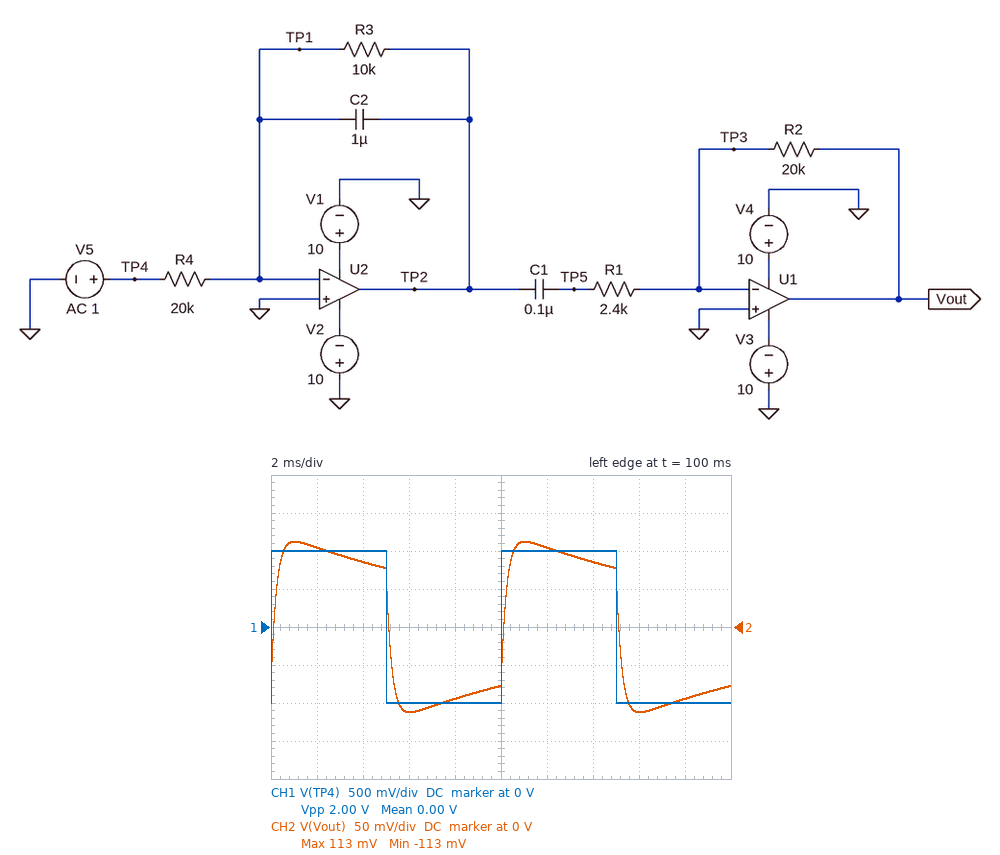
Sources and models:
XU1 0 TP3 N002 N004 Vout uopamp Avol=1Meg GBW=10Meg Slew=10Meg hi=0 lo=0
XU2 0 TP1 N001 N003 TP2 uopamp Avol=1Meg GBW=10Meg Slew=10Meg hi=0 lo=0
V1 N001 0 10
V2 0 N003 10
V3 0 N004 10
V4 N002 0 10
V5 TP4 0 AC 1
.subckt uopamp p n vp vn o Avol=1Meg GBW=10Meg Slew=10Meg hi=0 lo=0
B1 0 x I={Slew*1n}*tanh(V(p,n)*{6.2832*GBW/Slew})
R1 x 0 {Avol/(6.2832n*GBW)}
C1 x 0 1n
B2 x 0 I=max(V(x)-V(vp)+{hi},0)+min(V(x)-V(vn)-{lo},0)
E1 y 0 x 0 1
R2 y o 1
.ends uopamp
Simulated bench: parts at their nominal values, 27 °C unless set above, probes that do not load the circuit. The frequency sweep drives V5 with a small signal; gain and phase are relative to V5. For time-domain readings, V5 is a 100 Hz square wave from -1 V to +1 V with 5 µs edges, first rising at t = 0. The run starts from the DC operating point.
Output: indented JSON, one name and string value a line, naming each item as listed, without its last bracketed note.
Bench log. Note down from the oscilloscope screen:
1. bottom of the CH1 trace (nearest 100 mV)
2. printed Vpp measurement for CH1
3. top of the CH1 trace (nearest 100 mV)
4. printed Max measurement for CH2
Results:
{
  "bottom of the CH1 trace": "-1.0 V",
  "printed Vpp measurement for CH1": "2.00 V",
  "top of the CH1 trace": "1.0 V",
  "printed Max measurement for CH2": "113 mV"
}
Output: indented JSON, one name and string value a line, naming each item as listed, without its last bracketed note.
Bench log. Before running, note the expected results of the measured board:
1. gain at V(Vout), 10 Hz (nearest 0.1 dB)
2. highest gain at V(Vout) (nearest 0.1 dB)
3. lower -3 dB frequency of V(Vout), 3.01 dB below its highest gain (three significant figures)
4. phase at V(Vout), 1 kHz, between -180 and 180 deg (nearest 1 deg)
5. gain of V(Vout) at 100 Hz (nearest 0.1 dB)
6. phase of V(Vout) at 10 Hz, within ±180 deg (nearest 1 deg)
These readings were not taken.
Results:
{
  "gain at V(Vout), 10 Hz": "-25.5 dB",
  "highest gain at V(Vout)": "-20.2 dB",
  "lower -3 dB frequency of V(Vout), 3.01 dB below its highest gain": "15.2 Hz",
  "phase at V(Vout), 1 kHz, between -180 and 180 deg": "-56 deg",
  "gain of V(Vout) at 100 Hz": "-20.2 dB",
  "phase of V(Vout) at 10 Hz, within ±180 deg": "57 deg"
}
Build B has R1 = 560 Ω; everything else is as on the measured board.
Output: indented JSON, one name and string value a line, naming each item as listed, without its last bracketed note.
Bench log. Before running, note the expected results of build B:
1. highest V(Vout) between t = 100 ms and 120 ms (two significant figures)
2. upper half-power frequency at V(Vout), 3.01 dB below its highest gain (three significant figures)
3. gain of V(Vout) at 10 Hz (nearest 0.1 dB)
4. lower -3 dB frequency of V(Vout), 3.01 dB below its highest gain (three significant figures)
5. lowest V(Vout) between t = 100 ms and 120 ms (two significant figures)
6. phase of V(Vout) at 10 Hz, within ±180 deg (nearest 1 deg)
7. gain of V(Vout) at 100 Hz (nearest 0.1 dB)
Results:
{
  "highest V(Vout) between t = 100 ms and 120 ms": "120 mV",
  "upper half-power frequency at V(Vout), 3.01 dB below its highest gain": "2.90 kHz",
  "gain of V(Vout) at 10 Hz": "-25.5 dB",
  "lower -3 dB frequency of V(Vout), 3.01 dB below its highest gain": "15.7 Hz",
  "lowest V(Vout) between t = 100 ms and 120 ms": "-120 mV",
  "phase of V(Vout) at 10 Hz, within ±180 deg": "58 deg",
  "gain of V(Vout) at 100 Hz": "-20.1 dB"
}
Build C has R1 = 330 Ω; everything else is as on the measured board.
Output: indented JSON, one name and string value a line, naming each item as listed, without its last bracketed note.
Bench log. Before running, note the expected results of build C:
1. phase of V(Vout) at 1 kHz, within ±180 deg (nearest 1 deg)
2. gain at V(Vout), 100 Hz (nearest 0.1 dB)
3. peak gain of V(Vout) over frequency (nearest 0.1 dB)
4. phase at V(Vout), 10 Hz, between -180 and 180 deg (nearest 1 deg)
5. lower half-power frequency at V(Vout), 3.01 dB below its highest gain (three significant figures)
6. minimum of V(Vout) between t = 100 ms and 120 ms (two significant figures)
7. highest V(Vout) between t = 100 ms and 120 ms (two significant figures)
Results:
{
  "phase of V(Vout) at 1 kHz, within ±180 deg": "-11 deg",
  "gain at V(Vout), 100 Hz": "-20.1 dB",
  "peak gain of V(Vout) over frequency": "-20.0 dB",
  "phase at V(Vout), 10 Hz, between -180 and 180 deg": "58 deg",
  "lower half-power frequency at V(Vout), 3.01 dB below its highest gain": "15.8 Hz",
  "minimum of V(Vout) between t = 100 ms and 120 ms": "-120 mV",
  "highest V(Vout) between t = 100 ms and 120 ms": "120 mV"
}
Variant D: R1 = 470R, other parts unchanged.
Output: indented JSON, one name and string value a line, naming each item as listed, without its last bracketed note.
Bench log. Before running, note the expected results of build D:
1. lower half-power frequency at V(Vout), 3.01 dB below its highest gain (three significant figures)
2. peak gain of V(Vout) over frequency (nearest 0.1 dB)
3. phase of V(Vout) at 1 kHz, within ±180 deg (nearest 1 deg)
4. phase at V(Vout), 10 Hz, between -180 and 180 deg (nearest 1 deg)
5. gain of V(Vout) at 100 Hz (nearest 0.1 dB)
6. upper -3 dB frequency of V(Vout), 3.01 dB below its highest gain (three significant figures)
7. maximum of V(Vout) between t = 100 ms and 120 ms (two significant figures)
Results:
{
  "lower half-power frequency at V(Vout), 3.01 dB below its highest gain": "15.8 Hz",
  "peak gain of V(Vout) over frequency": "-20.0 dB",
  "phase of V(Vout) at 1 kHz, within ±180 deg": "-16 deg",
  "phase at V(Vout), 10 Hz, between -180 and 180 deg": "58 deg",
  "gain of V(Vout) at 100 Hz": "-20.1 dB",
  "upper -3 dB frequency of V(Vout), 3.01 dB below its highest gain": "3.47 kHz",
  "maximum of V(Vout) between t = 100 ms and 120 ms": "120 mV"
}
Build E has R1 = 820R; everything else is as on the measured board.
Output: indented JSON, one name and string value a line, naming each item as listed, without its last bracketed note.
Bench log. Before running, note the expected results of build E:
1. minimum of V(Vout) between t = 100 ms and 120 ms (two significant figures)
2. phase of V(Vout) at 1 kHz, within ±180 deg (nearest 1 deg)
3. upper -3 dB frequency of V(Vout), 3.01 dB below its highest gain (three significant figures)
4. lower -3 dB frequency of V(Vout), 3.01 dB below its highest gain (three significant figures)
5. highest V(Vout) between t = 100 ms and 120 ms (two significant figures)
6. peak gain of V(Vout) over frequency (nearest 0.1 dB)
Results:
{
  "minimum of V(Vout) between t = 100 ms and 120 ms": "-120 mV",
  "phase of V(Vout) at 1 kHz, within ±180 deg": "-26 deg",
  "upper -3 dB frequency of V(Vout), 3.01 dB below its highest gain": "1.98 kHz",
  "lower -3 dB frequency of V(Vout), 3.01 dB below its highest gain": "15.7 Hz",
  "highest V(Vout) between t = 100 ms and 120 ms": "120 mV",
  "peak gain of V(Vout) over frequency": "-20.1 dB"
}
